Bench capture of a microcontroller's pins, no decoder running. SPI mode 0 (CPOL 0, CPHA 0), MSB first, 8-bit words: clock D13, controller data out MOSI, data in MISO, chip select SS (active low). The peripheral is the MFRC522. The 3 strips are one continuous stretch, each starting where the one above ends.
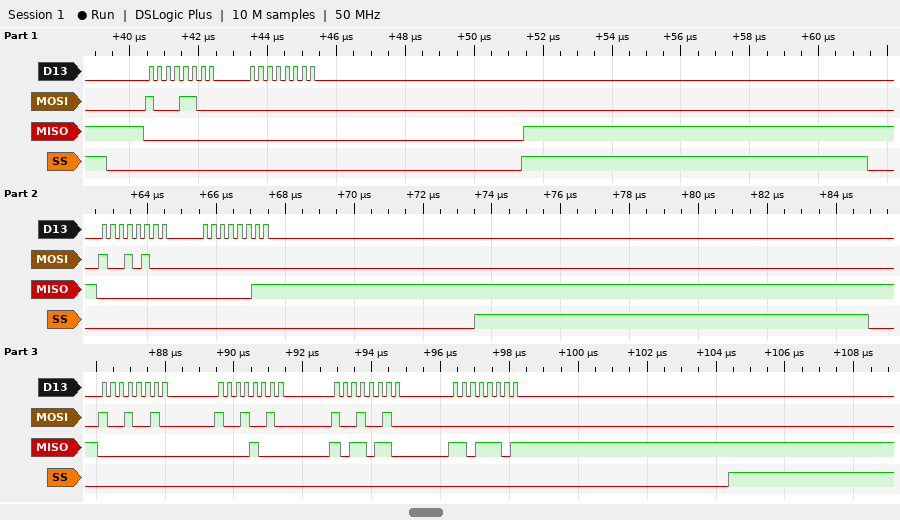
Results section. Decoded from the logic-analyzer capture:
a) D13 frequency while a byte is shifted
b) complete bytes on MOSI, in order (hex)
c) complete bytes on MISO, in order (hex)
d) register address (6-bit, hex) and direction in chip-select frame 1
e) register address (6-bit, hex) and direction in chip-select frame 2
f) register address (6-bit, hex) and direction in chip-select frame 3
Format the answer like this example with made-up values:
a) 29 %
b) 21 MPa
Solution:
a) 4 MHz
b) 8C 00 94 00 92 92 92 00
c) 00 00 00 03 00 08 B6 DD
d) 0x06 read
e) 0x0A read
f) 0x09 read
